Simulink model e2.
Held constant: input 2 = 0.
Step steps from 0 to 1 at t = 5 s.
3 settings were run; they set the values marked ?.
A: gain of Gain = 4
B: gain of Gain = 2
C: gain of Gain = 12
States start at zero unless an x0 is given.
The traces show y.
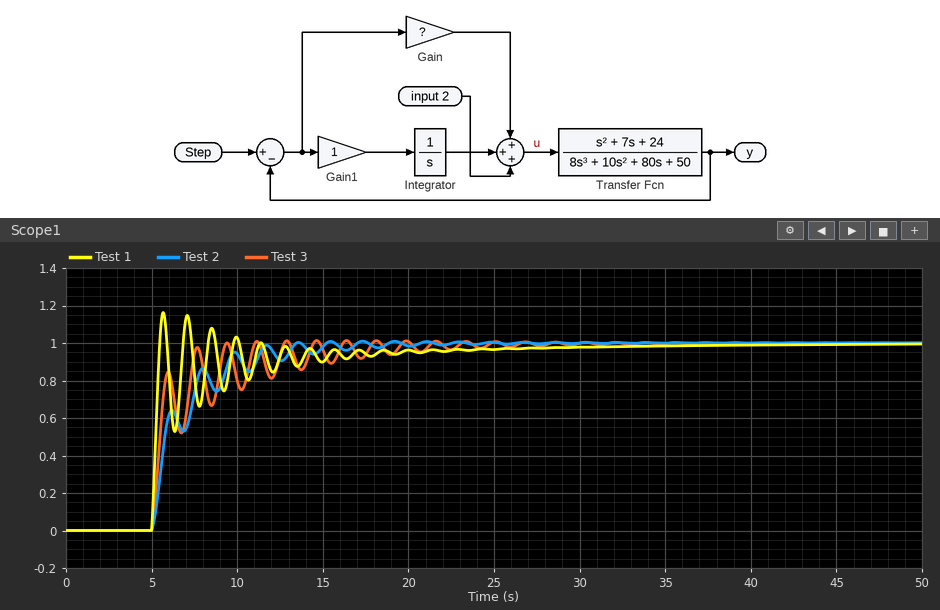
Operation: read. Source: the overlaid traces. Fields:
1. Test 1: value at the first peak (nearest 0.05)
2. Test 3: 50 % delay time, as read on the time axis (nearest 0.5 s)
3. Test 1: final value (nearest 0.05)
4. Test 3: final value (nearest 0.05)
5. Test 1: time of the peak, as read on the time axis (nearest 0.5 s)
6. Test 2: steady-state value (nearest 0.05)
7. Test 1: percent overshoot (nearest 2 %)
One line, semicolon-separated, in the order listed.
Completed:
1.15; 5.5 s; 1.00; 1.00; 5.5 s; 1.00; 16 %
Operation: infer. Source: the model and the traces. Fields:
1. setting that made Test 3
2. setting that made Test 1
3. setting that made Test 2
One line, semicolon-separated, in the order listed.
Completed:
A; C; B
